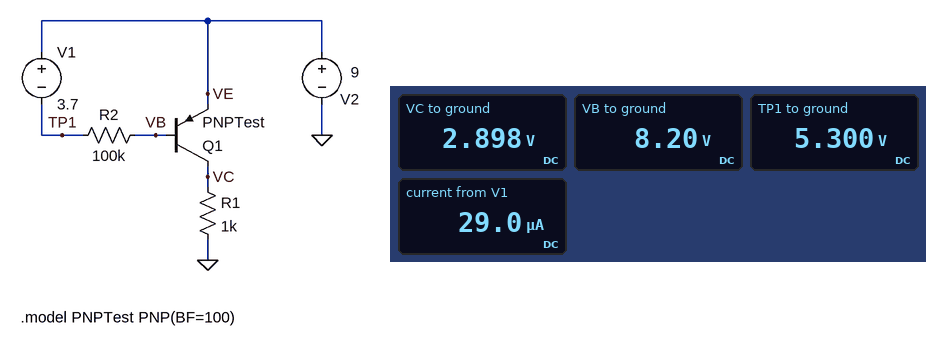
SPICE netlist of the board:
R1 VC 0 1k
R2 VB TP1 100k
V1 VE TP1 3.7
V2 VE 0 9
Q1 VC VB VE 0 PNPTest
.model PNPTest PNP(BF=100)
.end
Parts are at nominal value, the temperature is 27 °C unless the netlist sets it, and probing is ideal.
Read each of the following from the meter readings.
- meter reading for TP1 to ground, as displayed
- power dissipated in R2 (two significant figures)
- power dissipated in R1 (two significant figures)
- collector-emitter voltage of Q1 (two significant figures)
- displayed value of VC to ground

5.300 V
84 µW
8.4 mW
-6.1 V
2.898 V
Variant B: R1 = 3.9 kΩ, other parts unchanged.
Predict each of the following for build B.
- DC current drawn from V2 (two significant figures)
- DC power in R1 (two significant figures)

2.3 mA
20 mW
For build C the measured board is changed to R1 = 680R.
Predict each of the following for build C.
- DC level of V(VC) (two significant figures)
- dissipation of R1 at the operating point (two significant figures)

2.0 V
5.7 mW
